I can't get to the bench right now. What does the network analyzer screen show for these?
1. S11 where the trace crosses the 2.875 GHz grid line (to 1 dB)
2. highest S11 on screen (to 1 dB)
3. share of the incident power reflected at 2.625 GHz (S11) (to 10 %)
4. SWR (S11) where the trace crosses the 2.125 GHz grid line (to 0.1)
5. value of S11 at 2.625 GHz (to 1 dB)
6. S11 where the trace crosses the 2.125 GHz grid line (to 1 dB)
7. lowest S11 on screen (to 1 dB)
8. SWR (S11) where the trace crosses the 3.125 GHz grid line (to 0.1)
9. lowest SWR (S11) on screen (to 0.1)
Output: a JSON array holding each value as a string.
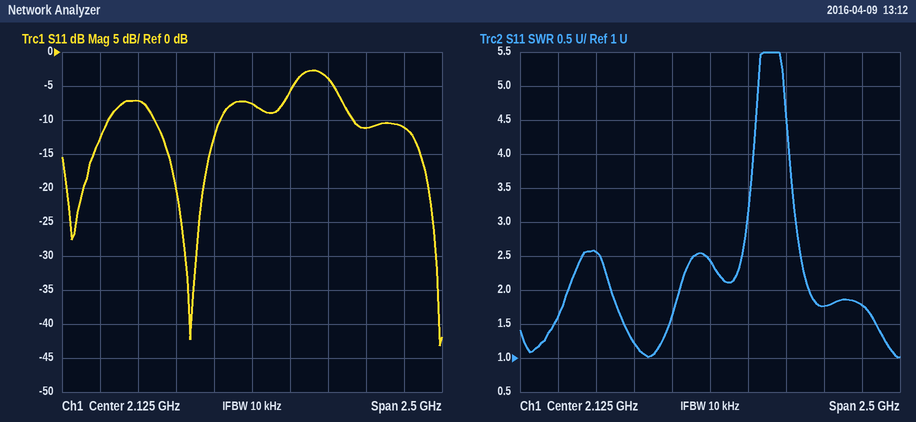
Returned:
["-11 dB", "-3 dB", "40 %", "2.4", "-4 dB", "-8 dB", "-43 dB", "1.8", "1.0"]
